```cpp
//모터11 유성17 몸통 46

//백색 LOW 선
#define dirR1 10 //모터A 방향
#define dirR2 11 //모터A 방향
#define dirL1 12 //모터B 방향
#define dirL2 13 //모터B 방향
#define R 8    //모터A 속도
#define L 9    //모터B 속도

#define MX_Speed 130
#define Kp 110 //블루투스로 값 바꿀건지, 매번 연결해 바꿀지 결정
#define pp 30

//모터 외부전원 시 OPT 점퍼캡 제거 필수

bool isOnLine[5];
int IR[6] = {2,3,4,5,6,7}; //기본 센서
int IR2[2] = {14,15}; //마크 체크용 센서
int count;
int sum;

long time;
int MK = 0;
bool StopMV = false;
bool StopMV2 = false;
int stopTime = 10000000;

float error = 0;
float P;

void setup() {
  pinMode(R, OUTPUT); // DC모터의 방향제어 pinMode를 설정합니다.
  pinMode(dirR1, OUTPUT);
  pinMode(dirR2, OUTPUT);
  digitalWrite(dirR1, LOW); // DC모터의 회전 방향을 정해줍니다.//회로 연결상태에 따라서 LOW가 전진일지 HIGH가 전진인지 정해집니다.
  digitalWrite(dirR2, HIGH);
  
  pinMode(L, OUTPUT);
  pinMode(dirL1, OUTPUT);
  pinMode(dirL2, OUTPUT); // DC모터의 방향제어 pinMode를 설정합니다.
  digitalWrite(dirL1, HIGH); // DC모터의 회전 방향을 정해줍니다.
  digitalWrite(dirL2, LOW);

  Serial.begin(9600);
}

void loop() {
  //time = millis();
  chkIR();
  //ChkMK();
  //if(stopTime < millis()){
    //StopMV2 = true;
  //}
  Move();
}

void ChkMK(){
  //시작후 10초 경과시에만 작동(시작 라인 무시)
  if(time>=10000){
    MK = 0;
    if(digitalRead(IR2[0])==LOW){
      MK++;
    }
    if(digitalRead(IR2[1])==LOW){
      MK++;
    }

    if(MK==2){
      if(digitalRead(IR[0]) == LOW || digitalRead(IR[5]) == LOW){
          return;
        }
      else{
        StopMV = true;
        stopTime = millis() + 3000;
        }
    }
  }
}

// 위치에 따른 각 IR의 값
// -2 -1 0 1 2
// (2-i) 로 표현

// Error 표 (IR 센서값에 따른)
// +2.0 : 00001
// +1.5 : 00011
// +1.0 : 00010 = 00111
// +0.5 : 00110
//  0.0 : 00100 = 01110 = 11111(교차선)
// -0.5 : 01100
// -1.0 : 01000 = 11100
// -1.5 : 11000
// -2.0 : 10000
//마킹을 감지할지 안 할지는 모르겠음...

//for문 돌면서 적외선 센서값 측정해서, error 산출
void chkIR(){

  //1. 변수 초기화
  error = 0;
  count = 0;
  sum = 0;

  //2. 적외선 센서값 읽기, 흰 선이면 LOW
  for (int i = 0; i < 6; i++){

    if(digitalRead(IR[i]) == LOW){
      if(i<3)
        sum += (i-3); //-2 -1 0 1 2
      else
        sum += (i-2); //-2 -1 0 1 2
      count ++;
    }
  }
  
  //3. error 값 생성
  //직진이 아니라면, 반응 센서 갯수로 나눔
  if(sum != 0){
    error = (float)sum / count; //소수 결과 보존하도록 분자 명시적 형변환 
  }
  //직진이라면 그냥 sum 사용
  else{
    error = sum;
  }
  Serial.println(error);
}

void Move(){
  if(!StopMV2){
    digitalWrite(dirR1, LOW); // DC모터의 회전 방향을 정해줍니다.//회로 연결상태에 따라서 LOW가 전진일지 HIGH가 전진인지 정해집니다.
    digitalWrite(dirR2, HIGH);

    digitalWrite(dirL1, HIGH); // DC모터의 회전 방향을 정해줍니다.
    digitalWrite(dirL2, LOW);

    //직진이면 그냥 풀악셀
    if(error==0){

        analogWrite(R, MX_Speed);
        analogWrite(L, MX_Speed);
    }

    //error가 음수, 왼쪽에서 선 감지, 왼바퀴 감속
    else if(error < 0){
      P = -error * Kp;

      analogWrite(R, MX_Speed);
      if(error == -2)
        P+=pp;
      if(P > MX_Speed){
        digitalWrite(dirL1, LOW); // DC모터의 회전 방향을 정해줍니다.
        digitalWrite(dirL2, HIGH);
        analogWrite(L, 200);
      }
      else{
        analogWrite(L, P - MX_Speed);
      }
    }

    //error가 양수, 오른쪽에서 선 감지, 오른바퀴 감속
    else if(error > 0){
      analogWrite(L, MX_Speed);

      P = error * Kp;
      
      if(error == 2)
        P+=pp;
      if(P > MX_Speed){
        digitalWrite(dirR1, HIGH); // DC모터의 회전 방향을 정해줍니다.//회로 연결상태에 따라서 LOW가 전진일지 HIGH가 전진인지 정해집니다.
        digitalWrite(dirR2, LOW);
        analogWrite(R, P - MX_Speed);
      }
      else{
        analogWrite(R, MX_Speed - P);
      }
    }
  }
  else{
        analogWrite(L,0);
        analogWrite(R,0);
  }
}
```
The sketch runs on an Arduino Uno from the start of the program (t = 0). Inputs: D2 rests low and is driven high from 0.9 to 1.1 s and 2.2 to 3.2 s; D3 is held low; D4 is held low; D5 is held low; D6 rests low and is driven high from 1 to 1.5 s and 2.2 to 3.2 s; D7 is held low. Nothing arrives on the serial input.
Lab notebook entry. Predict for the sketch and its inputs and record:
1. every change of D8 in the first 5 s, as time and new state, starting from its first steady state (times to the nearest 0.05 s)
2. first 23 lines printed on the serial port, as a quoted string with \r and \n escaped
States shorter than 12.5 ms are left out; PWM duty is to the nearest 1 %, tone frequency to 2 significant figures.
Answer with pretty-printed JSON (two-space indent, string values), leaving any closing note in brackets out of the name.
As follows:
{
  "every change of D8 in the first 5 s, as time and new state, starting from its first steady state": "0 s high; 0.9 s low; 1.1 s high; 2.2 s low; 3.2 s high",
  "first 23 lines printed on the serial port, as a quoted string with \\r and \\n escaped": "\"0.00\\r\\n0.00\\r\\n0.00\\r\\n0.00\\r\\n0.00\\r\\n0.00\\r\\n0.00\\r\\n0.00\\r\\n0.00\\r\\n0.00\\r\\n0.00\\r\\n0.00\\r\\n0.00\\r\\n0.00\\r\\n0.00\\r\\n0.00\\r\\n0.00\\r\\n0.00\\r\\n0.00\\r\\n0.00\\r\\n0.00\\r\\n0.00\\r\\n0.00\\r\\n\""
}
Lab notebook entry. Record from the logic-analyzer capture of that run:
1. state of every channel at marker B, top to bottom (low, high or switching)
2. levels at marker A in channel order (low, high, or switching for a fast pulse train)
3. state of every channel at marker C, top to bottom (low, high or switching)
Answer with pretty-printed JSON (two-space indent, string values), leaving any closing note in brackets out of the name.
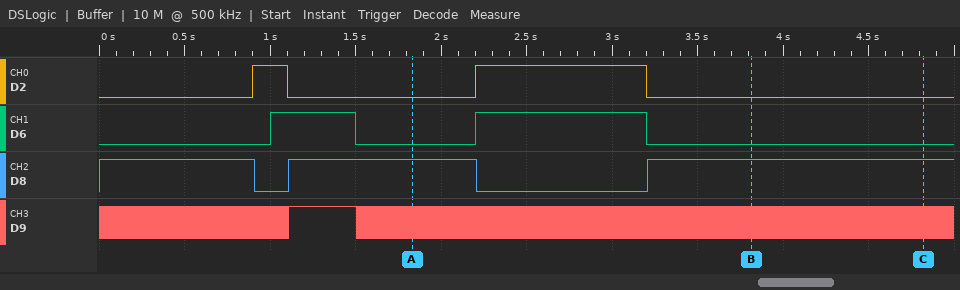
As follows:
{
  "state of every channel at marker B, top to bottom": "D2 low, D6 low, D8 high, D9 switching",
  "levels at marker A in channel order": "D2 low, D6 low, D8 high, D9 switching",
  "state of every channel at marker C, top to bottom": "D2 low, D6 low, D8 high, D9 switching"
}
